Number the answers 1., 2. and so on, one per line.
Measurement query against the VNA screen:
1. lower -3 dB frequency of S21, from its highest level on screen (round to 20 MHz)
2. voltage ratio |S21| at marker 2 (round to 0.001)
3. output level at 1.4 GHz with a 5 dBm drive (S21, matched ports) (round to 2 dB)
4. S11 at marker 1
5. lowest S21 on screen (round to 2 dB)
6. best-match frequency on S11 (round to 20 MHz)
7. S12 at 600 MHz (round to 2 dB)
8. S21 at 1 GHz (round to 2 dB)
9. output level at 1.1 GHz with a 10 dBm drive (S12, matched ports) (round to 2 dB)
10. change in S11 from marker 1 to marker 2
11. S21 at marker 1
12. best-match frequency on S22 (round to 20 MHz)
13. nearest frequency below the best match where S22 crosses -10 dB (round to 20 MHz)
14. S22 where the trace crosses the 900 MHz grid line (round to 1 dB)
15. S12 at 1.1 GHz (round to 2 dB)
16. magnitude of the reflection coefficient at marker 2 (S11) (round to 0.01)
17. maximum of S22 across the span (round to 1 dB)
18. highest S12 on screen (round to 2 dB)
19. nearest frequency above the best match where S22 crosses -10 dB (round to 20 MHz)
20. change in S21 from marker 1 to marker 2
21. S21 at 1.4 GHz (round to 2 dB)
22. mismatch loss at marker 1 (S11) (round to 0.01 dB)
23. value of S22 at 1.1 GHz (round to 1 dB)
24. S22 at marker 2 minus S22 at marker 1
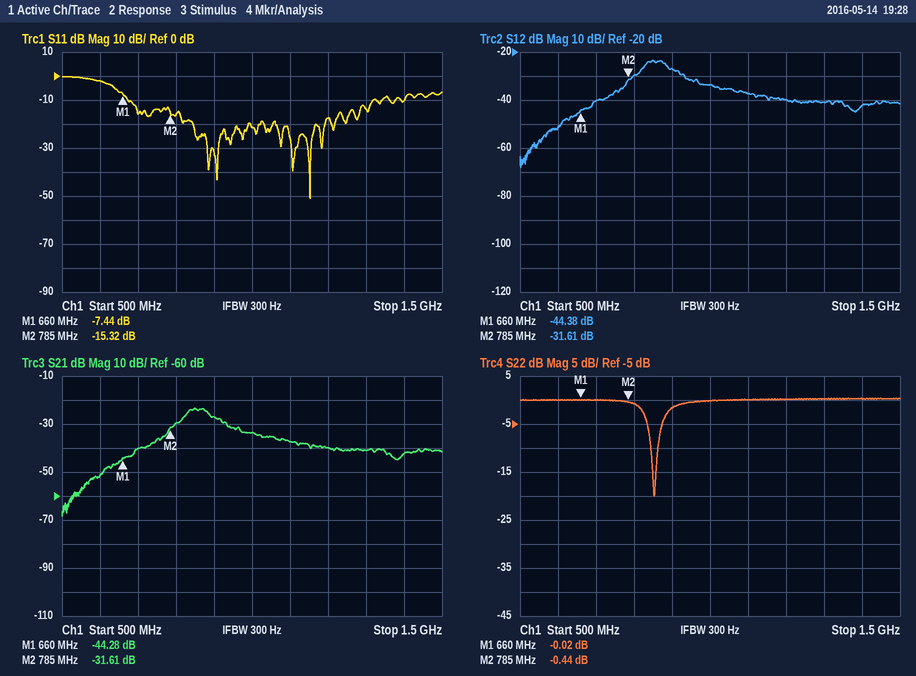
1. 820 MHz
2. 0.026
3. -38 dBm
4. -7.44 dB
5. -68 dB
6. 1.16 GHz
7. -52 dB
8. -34 dB
9. -28 dBm
10. -7.88 dB
11. -44.28 dB
12. 860 MHz
13. 840 MHz
14. -2 dB
15. -38 dB
16. 0.17
17. 0 dB
18. -24 dB
19. 860 MHz
20. 12.67 dB
21. -42 dB
22. 0.86 dB
23. 0 dB
24. -0.42 dB
